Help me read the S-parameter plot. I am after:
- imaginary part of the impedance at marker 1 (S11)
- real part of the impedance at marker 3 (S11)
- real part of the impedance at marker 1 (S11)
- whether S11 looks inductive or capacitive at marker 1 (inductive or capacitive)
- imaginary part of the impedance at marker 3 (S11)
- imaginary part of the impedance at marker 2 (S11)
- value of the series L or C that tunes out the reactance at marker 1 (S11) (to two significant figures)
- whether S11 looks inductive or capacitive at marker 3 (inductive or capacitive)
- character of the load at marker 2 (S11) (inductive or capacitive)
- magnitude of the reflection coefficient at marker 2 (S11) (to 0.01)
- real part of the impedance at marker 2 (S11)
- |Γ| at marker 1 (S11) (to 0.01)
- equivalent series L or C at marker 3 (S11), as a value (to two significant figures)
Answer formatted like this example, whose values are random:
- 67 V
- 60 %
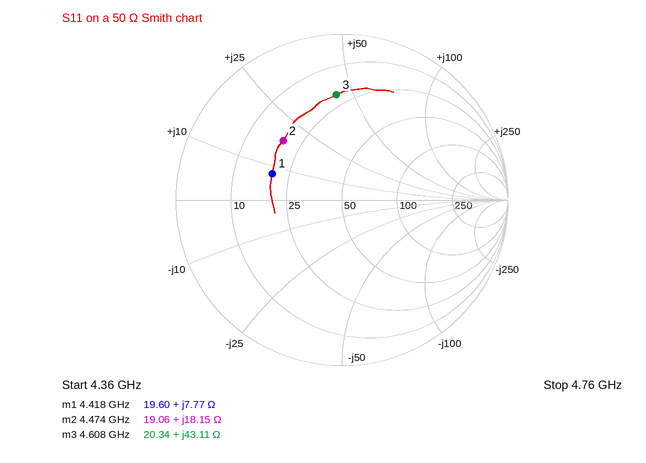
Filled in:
- +7.77 Ω
- 20.34 Ω
- 19.60 Ω
- inductive
- +43.11 Ω
- +18.15 Ω
- 4.6 pF
- inductive
- inductive
- 0.50
- 19.06 Ω
- 0.45
- 1.5 nH
